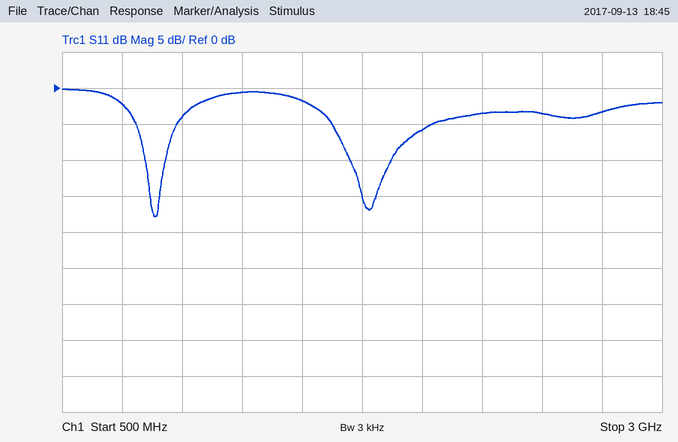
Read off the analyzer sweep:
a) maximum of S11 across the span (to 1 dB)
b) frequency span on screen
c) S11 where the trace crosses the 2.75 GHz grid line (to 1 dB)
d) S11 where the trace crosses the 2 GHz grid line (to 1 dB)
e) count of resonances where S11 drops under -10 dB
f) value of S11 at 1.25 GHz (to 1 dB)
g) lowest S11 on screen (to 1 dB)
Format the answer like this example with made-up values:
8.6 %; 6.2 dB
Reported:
0 dB; 2.5 GHz; -3 dB; -6 dB; 2; -1 dB; -18 dB
